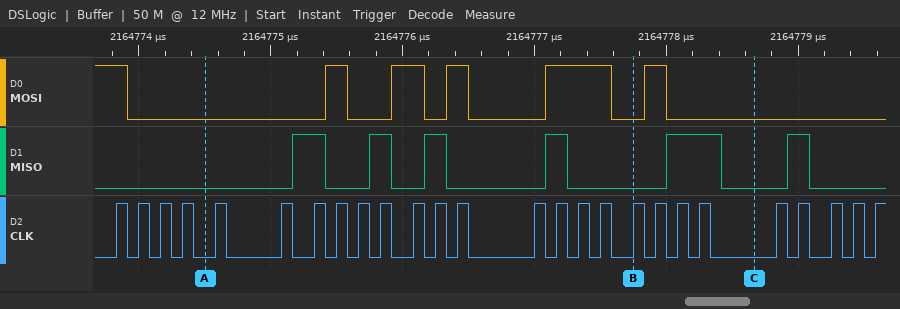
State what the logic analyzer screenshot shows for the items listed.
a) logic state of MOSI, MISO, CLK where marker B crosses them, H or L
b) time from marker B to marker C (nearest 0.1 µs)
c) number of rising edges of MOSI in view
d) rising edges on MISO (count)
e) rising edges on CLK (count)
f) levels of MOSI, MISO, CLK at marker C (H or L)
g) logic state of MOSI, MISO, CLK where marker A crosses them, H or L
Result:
MOSI=L, MISO=L, CLK=H
0.9 µs
5
6
26
MOSI=L, MISO=L, CLK=L
MOSI=L, MISO=L, CLK=L
